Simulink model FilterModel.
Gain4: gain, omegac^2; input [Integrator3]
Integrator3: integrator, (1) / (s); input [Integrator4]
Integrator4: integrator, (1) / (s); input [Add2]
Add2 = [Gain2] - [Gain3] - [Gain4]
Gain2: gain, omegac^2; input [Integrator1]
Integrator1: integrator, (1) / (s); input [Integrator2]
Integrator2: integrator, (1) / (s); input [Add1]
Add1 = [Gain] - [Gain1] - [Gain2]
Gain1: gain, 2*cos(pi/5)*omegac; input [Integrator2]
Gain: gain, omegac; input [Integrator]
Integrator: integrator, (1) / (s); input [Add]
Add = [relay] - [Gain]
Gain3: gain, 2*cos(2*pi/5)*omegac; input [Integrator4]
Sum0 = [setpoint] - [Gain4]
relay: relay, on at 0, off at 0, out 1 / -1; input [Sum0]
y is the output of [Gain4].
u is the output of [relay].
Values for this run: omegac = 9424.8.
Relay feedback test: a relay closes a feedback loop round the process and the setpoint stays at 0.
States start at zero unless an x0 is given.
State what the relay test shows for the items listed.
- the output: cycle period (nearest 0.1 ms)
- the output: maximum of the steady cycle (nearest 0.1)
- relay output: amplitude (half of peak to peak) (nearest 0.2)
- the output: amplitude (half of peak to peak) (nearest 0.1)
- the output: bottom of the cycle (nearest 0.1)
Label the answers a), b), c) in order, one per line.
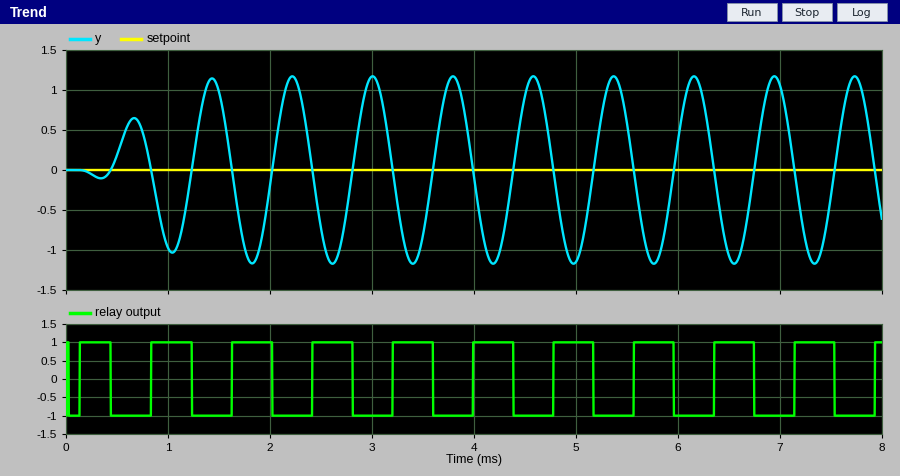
a) 0.8 ms
b) 1.2
c) 1.0
d) 1.2
e) -1.2
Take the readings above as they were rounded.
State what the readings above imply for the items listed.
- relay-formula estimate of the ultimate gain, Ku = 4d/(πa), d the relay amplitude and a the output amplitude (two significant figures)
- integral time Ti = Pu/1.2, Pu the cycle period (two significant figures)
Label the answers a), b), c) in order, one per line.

a) 1.1
b) 0.67 ms
